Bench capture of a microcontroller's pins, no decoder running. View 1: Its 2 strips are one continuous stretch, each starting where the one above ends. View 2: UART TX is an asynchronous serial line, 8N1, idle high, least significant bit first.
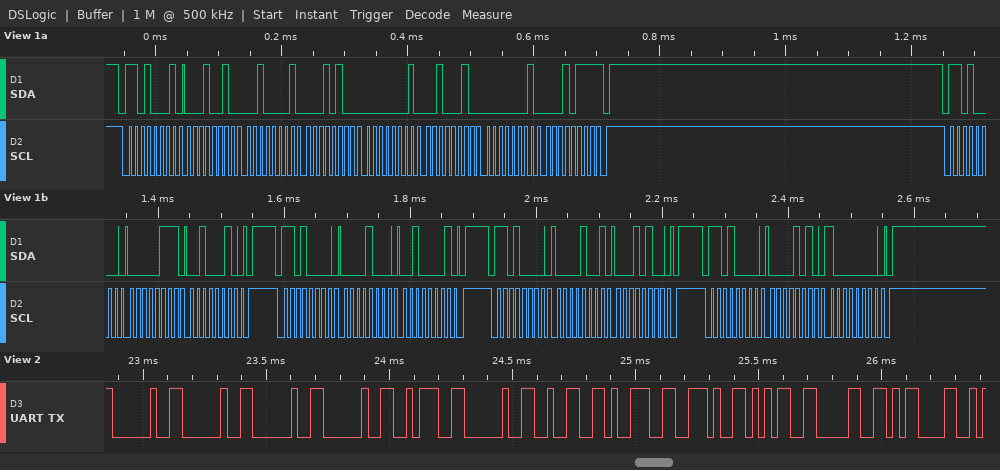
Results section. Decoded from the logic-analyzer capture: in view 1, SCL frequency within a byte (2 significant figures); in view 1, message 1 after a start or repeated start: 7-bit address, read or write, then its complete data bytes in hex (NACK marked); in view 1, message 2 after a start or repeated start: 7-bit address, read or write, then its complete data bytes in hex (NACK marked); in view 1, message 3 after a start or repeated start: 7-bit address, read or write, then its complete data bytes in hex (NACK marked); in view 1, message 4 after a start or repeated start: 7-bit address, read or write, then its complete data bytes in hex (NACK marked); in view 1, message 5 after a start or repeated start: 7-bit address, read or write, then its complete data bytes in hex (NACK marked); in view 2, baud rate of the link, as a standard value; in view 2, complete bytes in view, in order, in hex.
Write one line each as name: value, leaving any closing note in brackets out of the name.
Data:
in view 1, SCL frequency within a byte: 100 kHz
in view 1, message 1 after a start or repeated start: 7-bit address, read or write, then its complete data bytes in hex: 0x68 read: 12 21 14 01 22 01 17 NACK
in view 1, message 2 after a start or repeated start: 7-bit address, read or write, then its complete data bytes in hex: 0x68 write: 07 22
in view 1, message 3 after a start or repeated start: 7-bit address, read or write, then its complete data bytes in hex: 0x68 write: 08 21
in view 1, message 4 after a start or repeated start: 7-bit address, read or write, then its complete data bytes in hex: 0x68 write: 09 14
in view 1, message 5 after a start or repeated start: 7-bit address, read or write, then its complete data bytes in hex: 0x68 write: 0A 80
in view 2, baud rate of the link, as a standard value: 38400 baud
in view 2, complete bytes in view, in order, in hex: 20 20 20 20 3A 20 32 39 2E 35 30 0D
